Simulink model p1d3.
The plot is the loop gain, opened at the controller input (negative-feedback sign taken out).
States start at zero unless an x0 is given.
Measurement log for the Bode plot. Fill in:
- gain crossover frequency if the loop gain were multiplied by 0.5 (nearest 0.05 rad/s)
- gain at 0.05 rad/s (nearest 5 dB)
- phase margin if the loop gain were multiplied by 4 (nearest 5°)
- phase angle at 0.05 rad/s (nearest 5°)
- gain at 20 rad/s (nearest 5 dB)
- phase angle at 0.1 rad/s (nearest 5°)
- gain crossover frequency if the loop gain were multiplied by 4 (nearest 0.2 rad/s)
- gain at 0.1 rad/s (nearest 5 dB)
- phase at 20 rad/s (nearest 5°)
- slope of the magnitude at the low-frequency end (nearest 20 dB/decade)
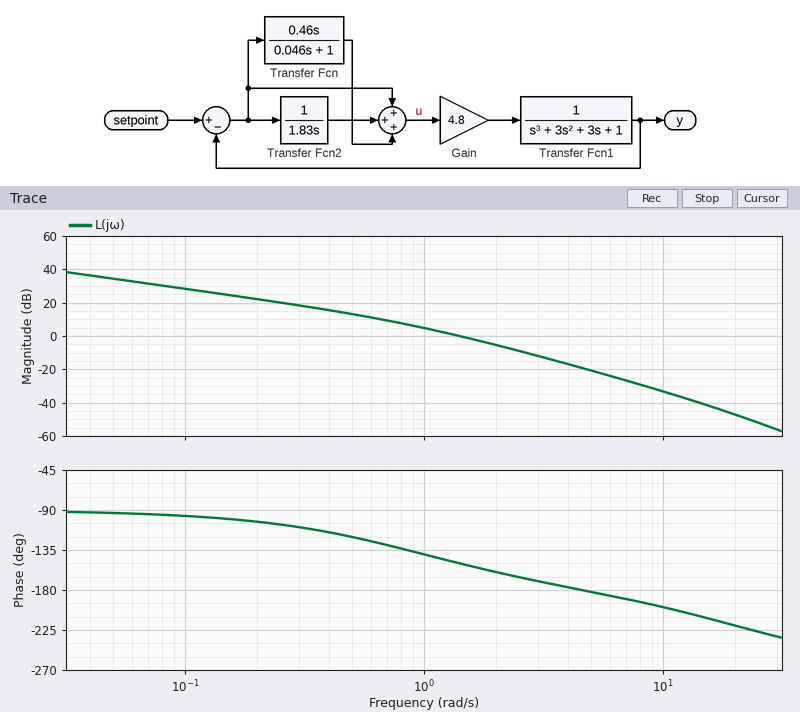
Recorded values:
0.90 rad/s
35 dB
10°
-95°
-45 dB
-95°
3.0 rad/s
30 dB
-220°
-20 dB/decade
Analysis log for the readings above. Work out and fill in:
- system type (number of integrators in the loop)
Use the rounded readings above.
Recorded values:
1
